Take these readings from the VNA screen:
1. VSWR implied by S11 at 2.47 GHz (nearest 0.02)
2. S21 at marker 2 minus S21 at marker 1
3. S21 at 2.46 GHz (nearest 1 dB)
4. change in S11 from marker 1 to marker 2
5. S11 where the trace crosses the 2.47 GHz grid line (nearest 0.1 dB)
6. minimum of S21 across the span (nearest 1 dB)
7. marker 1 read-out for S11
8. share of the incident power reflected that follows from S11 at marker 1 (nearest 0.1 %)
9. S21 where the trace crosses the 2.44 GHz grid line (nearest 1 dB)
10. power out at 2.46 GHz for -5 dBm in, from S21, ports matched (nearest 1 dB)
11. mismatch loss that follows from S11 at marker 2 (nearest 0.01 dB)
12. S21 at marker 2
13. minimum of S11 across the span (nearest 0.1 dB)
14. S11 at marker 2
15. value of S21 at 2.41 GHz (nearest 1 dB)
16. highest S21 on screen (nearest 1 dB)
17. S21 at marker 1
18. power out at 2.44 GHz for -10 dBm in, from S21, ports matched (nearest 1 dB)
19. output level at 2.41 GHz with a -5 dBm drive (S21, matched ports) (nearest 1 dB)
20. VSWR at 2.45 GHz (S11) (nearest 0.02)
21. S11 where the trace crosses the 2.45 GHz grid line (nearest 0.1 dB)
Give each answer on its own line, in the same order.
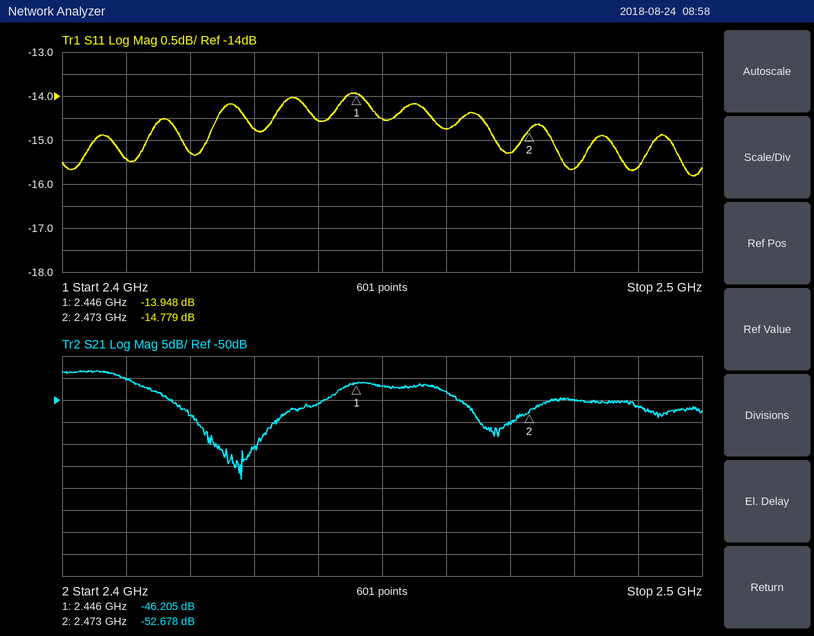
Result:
1.42
-6.473 dB
-48 dB
-0.831 dB
-15.3 dB
-68 dB
-13.948 dB
4.0 %
-51 dB
-53 dBm
0.15 dB
-52.678 dB
-15.8 dB
-14.779 dB
-45 dB
-43 dB
-46.205 dB
-61 dBm
-50 dBm
1.46
-14.5 dB
